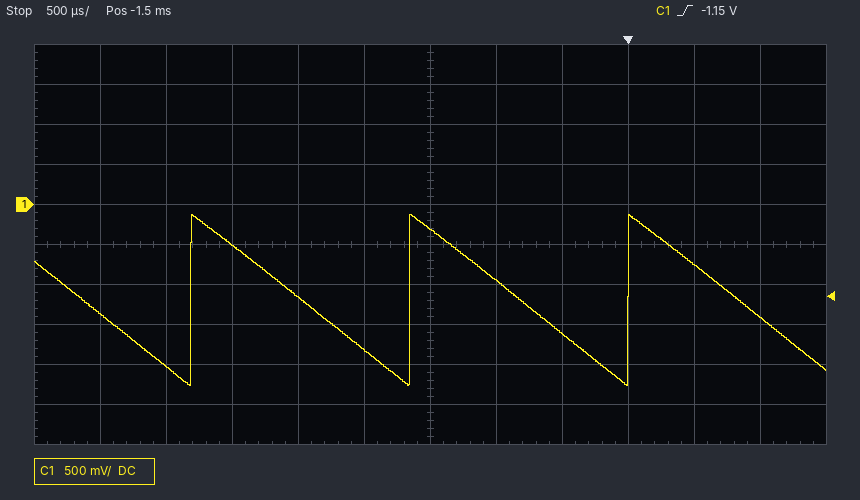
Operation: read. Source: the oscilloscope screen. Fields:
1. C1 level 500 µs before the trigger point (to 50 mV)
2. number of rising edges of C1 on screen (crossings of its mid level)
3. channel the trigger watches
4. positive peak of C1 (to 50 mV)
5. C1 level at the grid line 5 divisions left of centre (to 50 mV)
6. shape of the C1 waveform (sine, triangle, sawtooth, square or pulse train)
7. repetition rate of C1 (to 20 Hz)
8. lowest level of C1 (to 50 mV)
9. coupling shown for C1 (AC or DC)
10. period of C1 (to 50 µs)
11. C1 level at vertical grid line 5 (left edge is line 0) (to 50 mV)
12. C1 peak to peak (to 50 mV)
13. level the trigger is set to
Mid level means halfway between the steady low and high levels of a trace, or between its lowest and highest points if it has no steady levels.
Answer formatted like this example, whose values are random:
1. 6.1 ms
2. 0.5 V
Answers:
1. -1.60 V
2. 3
3. C1
4. -100 mV
5. -1.35 V
6. sawtooth
7. 600 Hz
8. -2.25 V
9. DC
10. 1.65 ms
11. -1.80 V
12. 2.15 V
13. -1.15 V
